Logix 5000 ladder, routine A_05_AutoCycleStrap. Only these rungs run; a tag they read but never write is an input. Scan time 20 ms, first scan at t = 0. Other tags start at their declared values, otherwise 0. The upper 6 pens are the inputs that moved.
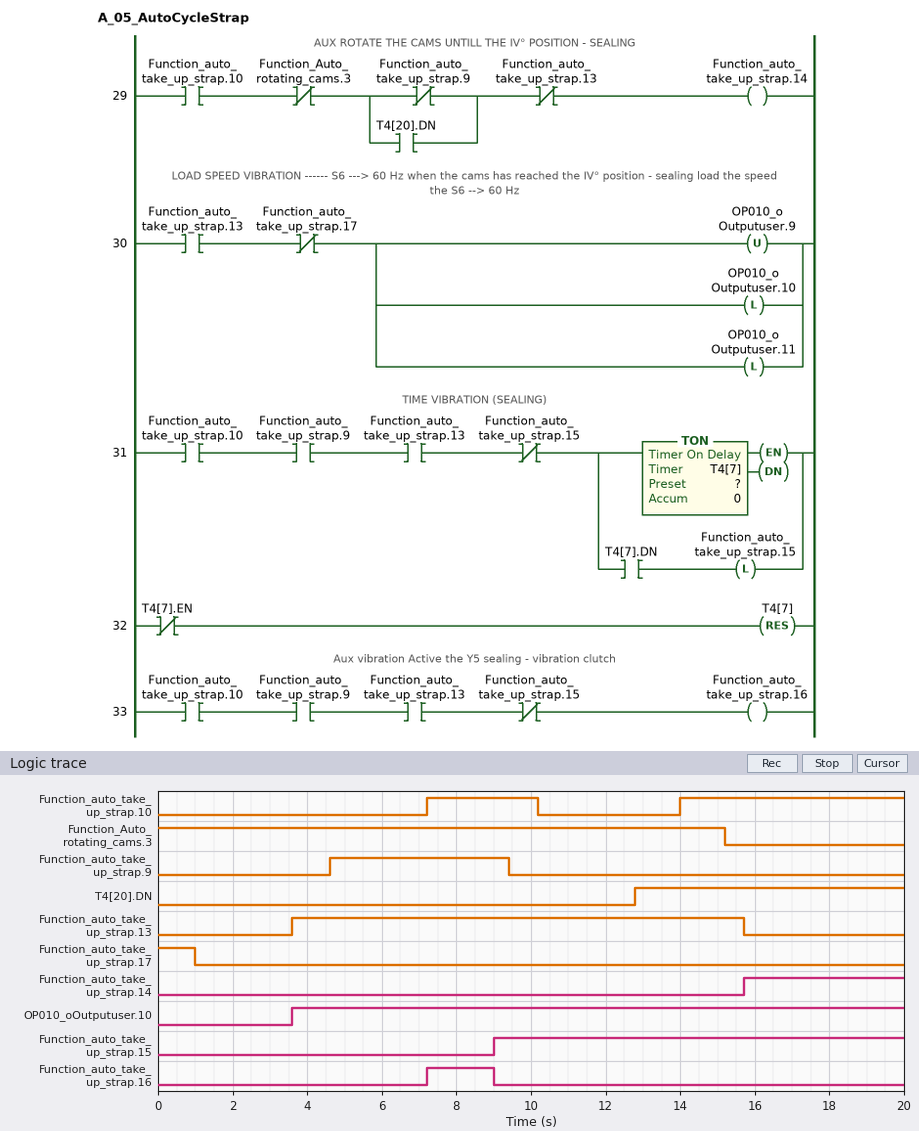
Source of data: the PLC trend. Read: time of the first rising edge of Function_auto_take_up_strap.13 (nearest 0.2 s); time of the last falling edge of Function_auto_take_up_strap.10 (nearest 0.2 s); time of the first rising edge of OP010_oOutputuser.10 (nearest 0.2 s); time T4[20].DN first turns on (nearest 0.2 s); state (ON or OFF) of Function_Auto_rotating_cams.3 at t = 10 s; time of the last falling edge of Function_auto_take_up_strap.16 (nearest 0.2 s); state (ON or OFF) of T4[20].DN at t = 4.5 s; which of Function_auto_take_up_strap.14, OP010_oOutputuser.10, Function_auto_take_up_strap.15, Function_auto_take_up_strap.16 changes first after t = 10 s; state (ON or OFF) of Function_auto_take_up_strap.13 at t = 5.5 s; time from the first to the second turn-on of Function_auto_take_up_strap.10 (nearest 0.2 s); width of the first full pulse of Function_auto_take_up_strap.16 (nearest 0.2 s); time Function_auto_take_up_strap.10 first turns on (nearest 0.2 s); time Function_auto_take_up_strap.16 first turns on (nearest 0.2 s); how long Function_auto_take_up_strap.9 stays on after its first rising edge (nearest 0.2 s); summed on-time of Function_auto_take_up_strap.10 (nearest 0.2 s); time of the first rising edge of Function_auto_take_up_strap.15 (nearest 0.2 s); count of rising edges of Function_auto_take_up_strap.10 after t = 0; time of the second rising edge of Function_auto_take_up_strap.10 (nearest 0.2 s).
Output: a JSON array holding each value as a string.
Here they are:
["3.6 s", "10.2 s", "3.6 s", "12.8 s", "ON", "9.0 s", "OFF", "Function_auto_take_up_strap.14", "ON", "6.8 s", "1.8 s", "7.2 s", "7.2 s", "4.8 s", "9.0 s", "9.0 s", "2", "14.0 s"]
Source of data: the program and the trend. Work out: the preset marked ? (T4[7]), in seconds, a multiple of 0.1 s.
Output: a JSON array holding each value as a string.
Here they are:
["1.8 s"]
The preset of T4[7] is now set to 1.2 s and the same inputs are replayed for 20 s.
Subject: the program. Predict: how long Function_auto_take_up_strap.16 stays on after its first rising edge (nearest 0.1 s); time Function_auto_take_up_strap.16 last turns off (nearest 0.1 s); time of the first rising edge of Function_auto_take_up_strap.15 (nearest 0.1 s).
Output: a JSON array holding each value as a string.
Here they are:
["1.2 s", "8.4 s", "8.4 s"]
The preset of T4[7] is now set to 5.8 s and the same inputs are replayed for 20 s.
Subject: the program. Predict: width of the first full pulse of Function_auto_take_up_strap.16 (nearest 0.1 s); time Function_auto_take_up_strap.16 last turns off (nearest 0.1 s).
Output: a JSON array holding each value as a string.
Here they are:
["2.2 s", "9.4 s"]
